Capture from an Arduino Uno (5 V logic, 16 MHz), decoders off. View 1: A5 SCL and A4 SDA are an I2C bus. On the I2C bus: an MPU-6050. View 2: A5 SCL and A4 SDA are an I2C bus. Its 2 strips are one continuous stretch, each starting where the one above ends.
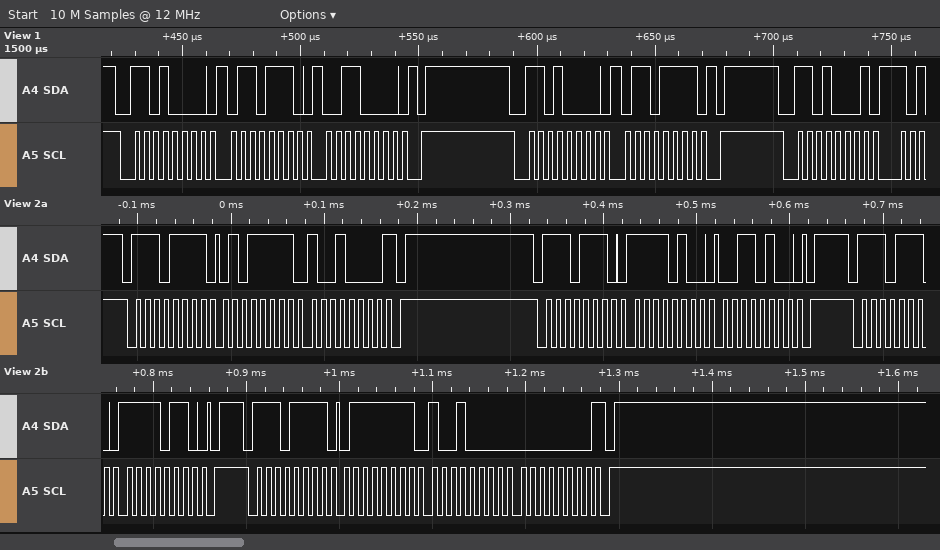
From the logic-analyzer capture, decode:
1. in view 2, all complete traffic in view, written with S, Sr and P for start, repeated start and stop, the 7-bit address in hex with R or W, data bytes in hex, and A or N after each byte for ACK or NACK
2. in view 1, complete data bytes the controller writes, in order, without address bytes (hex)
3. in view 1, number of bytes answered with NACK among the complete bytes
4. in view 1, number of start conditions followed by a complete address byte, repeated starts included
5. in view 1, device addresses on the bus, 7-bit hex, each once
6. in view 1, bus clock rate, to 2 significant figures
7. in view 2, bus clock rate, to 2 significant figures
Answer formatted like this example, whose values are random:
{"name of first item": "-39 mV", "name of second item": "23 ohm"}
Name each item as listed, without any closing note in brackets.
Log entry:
{"in view 2, all complete traffic in view, written with S, Sr and P for start, repeated start and stop, the 7-bit address in hex with R or W, data bytes in hex, and A or N after each byte for ACK or NACK": "S 77R A 5F A 90 N P S 77W A F4 A 34 A P S 77W A F6 A P S 77R A 7F A 90 A 00 N P", "in view 1, complete data bytes the controller writes, in order, without address bytes": "6E 30 6F", "in view 1, number of bytes answered with NACK among the complete bytes": "0", "in view 1, number of start conditions followed by a complete address byte, repeated starts included": "3", "in view 1, device addresses on the bus, 7-bit hex, each once": "0x68", "in view 1, bus clock rate, to 2 significant figures": "250 kHz", "in view 2, bus clock rate, to 2 significant figures": "100 kHz"}
